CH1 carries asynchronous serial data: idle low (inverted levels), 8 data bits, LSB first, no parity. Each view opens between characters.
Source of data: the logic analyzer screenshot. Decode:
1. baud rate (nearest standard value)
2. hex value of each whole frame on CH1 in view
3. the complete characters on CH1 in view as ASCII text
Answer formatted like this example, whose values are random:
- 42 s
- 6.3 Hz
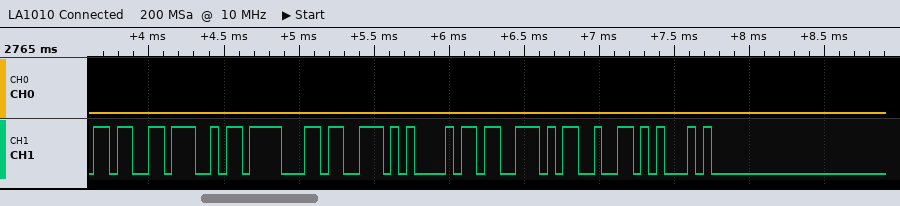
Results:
- 19200 baud
- 32, 2C, 38, 46, 2F, 46, 36, 5D
- "2,8F/F6]"
